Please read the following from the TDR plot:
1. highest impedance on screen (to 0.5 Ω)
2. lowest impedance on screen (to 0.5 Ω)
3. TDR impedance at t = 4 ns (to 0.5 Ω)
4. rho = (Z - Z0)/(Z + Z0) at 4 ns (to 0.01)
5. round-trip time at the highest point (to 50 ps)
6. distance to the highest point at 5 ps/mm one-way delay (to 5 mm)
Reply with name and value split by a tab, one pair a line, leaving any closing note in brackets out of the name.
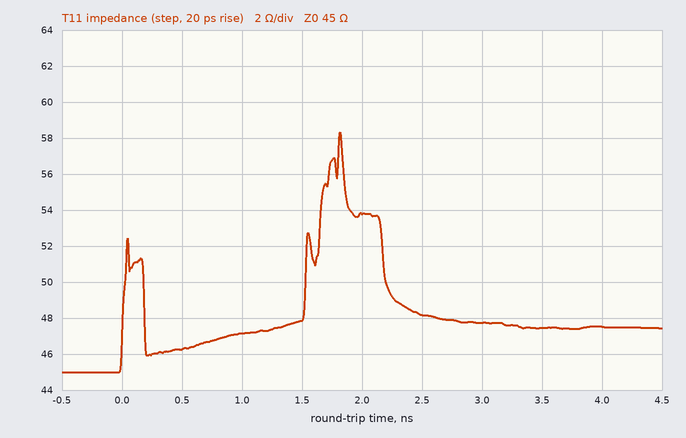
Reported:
highest impedance on screen	58.5 Ω
lowest impedance on screen	45.0 Ω
TDR impedance at t = 4 ns	47.5 Ω
rho = (Z - Z0)/(Z + Z0) at 4 ns	+0.03
round-trip time at the highest point	1.80 ns
distance to the highest point at 5 ps/mm one-way delay	180 mm
